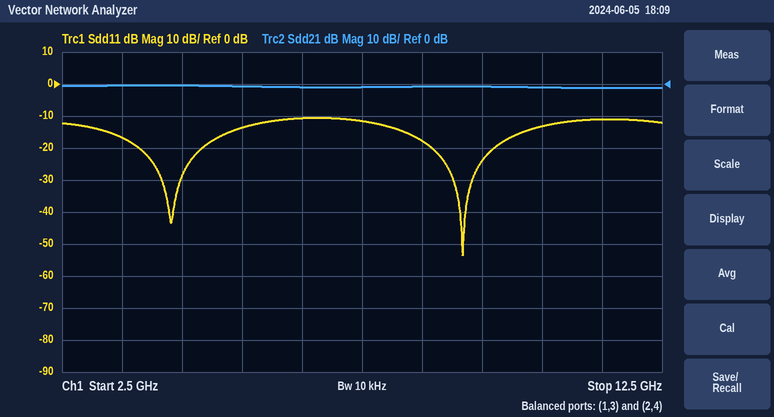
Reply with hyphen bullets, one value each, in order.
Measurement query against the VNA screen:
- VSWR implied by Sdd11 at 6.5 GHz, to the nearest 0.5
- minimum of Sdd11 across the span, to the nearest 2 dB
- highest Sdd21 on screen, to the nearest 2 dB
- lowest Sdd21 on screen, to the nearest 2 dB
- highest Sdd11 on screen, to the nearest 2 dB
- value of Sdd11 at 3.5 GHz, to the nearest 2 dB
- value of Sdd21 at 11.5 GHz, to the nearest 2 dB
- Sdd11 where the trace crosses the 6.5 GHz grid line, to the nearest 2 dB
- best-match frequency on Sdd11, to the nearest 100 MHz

- 2.0
- -54 dB
- 0 dB
- -2 dB
- -10 dB
- -16 dB
- -2 dB
- -10 dB
- 9.2 GHz
